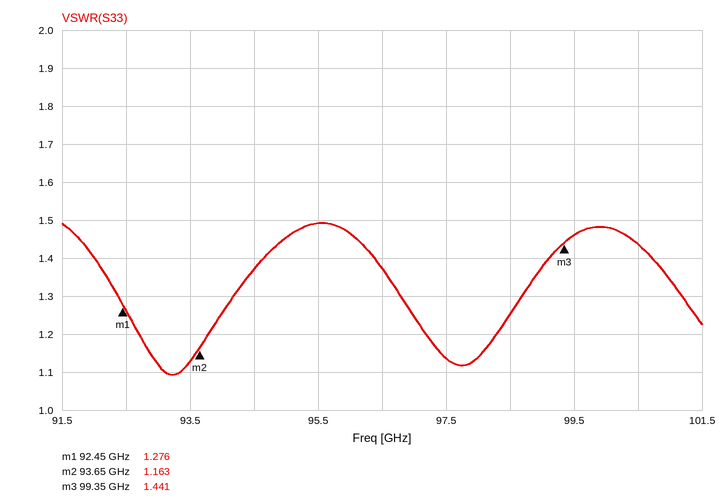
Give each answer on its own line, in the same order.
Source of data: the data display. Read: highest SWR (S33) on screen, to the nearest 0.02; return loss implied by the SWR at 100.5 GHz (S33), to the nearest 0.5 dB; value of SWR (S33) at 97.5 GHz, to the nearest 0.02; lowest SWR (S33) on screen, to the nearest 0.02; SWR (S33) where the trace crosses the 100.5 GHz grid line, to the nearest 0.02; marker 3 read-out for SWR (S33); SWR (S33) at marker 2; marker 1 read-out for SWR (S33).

1.50
15.0 dB
1.14
1.10
1.44
1.441
1.163
1.276
